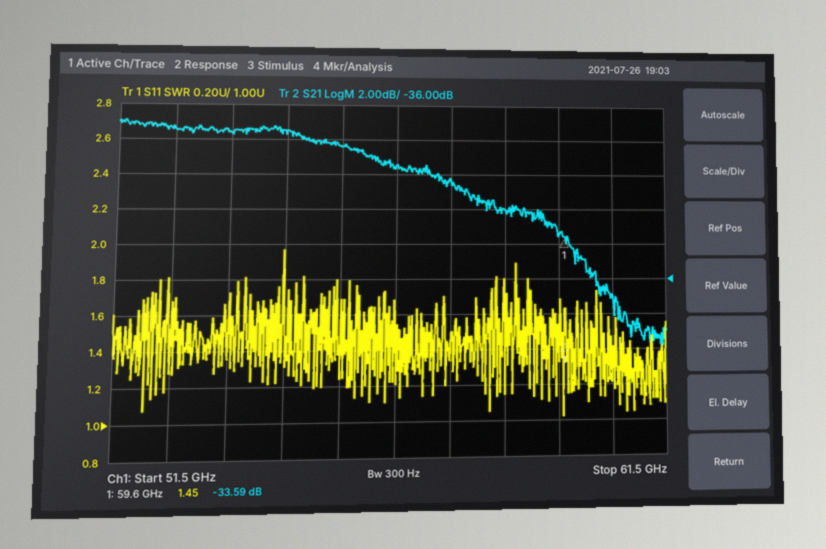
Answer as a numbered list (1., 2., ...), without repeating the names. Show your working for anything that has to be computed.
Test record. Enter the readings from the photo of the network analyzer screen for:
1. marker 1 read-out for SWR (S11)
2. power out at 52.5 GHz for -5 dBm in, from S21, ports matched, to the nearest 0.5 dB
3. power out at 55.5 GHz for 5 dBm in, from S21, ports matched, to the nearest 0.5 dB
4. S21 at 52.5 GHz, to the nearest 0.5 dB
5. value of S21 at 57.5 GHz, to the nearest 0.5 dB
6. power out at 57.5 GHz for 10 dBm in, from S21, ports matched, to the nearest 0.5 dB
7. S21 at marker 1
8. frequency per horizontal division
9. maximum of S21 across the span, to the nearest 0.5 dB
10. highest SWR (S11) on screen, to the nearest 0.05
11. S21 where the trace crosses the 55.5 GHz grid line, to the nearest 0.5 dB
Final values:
1. 1.45
2. -5 dBm + (-27.5 dB) = -32.5 dBm
3. 5 dBm + (-28.5 dB) = -23.5 dBm
4. -27.5 dB
5. -30.5 dB
6. 10 dBm + (-30.5 dB) = -20.5 dBm
7. -33.59 dB
8. 1 GHz
9. -27.0 dB
10. 1.95
11. -28.5 dB
